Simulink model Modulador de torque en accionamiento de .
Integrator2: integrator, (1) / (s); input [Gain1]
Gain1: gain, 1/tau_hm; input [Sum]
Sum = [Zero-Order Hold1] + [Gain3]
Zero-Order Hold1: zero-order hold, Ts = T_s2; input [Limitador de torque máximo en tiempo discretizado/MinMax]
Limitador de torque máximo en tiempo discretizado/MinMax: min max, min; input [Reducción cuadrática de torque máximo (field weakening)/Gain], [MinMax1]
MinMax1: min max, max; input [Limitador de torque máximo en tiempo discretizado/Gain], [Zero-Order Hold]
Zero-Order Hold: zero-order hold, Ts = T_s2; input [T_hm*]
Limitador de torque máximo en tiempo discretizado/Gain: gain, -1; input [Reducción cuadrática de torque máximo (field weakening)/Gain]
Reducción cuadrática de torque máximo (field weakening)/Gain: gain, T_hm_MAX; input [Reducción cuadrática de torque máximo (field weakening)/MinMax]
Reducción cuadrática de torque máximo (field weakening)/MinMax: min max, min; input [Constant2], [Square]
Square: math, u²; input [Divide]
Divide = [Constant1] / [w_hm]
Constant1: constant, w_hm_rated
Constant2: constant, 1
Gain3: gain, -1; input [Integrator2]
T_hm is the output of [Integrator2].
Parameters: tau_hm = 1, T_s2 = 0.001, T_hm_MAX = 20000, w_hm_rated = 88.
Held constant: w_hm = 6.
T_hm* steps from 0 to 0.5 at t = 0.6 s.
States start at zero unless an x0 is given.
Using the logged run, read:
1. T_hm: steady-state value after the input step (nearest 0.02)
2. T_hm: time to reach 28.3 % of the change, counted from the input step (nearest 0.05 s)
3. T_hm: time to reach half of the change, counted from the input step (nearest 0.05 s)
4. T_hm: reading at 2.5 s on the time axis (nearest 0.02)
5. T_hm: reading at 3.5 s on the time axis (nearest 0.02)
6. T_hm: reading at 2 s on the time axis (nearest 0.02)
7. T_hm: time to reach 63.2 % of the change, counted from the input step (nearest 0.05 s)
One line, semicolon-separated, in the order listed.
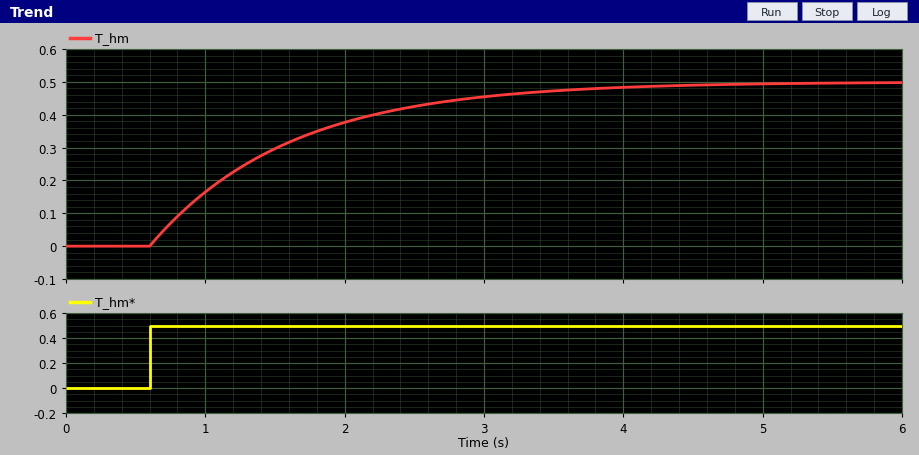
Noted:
0.50; 0.35 s; 0.70 s; 0.42; 0.48; 0.38; 1.00 s
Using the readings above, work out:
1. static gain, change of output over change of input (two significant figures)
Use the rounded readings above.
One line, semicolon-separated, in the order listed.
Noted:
1.0
